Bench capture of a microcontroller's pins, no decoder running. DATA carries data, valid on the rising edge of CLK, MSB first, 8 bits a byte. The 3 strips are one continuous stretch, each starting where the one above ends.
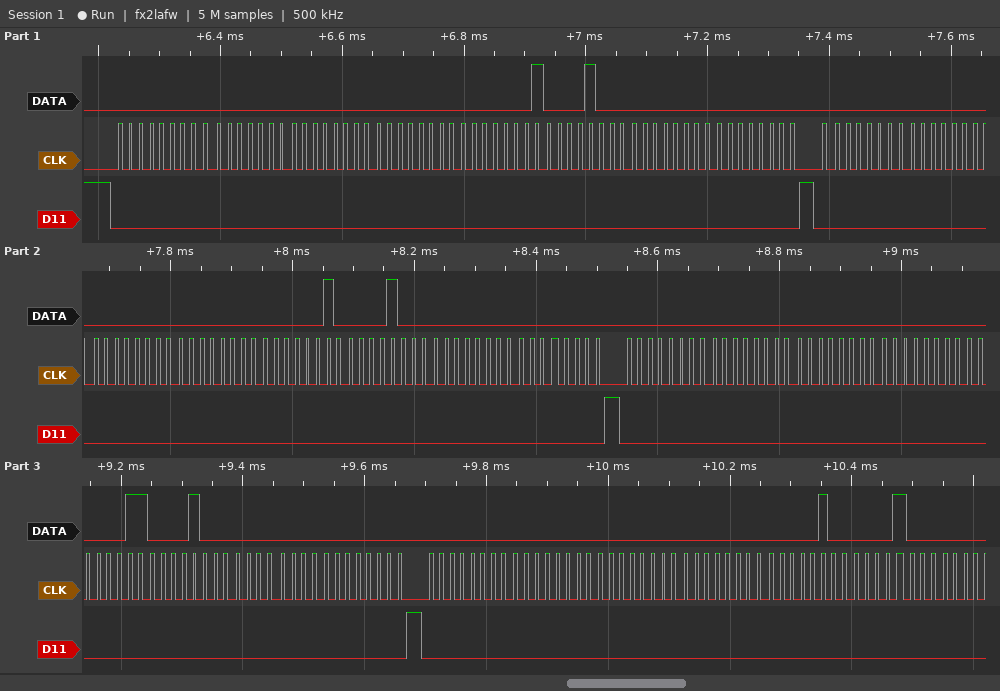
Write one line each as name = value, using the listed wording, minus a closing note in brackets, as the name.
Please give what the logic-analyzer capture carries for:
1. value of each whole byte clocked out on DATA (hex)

value of each whole byte clocked out on DATA = 00 00 00 00 01 08 00 00 00 00 00 00 02 08 00 00 00 00 00 00 03 08 00 00 00 00 00 00 04 08
